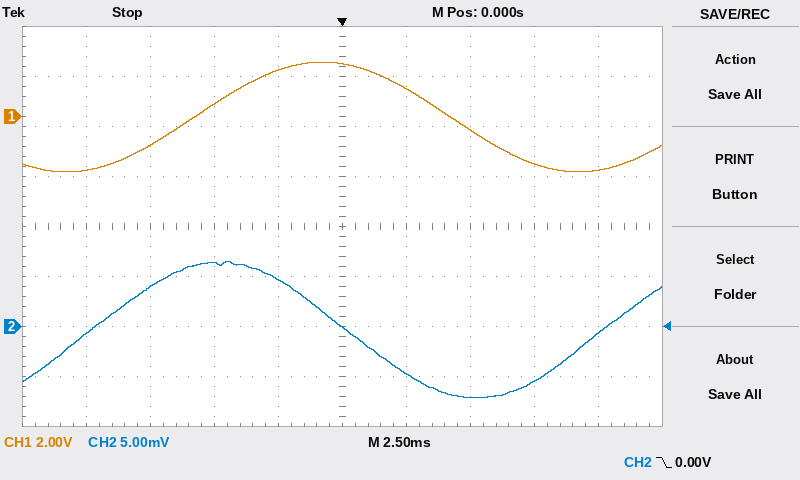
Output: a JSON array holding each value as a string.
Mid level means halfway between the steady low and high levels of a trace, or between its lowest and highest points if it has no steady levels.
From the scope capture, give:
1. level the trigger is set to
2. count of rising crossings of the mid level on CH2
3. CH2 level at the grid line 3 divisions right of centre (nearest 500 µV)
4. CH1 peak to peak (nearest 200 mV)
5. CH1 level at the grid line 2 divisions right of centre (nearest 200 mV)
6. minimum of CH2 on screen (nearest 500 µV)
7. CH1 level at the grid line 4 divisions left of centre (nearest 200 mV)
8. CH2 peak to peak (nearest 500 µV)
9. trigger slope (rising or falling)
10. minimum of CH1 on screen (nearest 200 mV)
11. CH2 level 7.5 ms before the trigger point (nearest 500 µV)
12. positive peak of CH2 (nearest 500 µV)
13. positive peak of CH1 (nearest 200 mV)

["0.00 V", "2", "-5.5 mV", "4.4 V", "-600 mV", "-7.0 mV", "-2.2 V", "13.5 mV", "falling", "-2.2 V", "4.0 mV", "6.5 mV", "2.2 V"]
